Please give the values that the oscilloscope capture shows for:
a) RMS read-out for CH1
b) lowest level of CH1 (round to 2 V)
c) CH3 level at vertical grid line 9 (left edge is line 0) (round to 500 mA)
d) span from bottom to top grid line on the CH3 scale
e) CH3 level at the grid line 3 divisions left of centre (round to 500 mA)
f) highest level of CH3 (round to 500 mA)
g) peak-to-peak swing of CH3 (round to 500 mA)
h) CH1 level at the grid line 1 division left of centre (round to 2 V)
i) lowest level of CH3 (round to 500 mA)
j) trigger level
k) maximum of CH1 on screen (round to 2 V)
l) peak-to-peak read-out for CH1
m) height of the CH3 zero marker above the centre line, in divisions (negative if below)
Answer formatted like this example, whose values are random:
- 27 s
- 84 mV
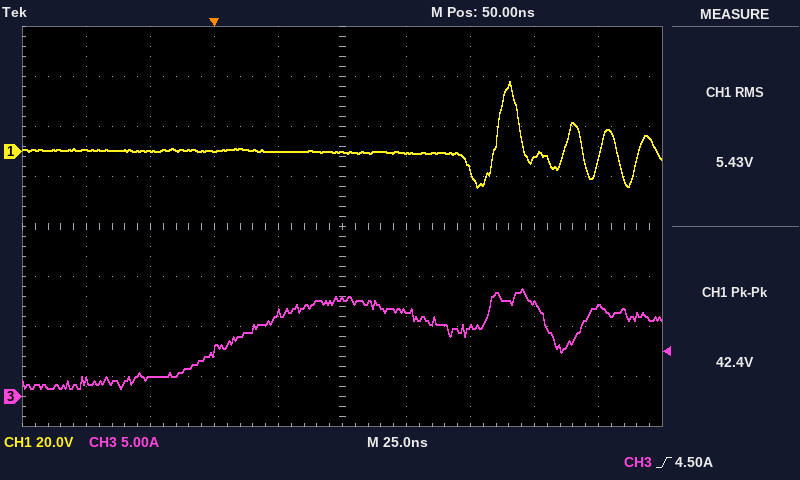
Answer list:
- 5.43 V
- -14 V
- 9.0 A
- 40 A
- 2.0 A
- 11.0 A
- 10.0 A
- 0 V
- 1.0 A
- 4.50 A
- 28 V
- 42.4 V
- -3.4 div
